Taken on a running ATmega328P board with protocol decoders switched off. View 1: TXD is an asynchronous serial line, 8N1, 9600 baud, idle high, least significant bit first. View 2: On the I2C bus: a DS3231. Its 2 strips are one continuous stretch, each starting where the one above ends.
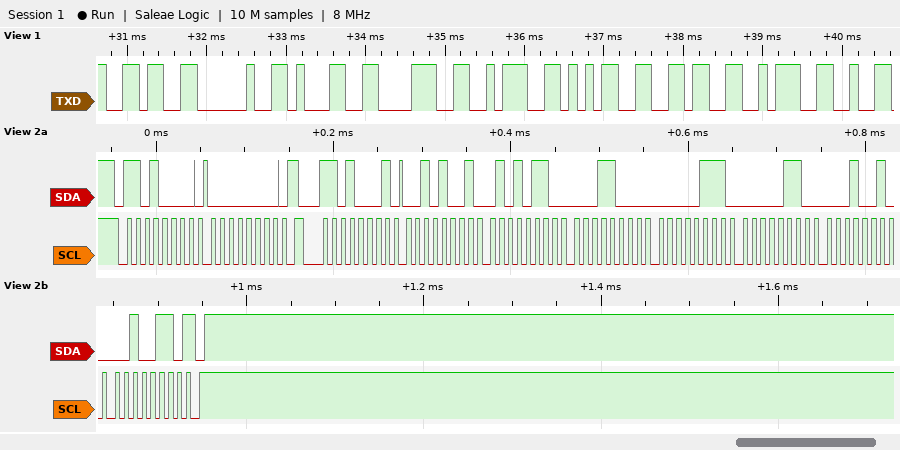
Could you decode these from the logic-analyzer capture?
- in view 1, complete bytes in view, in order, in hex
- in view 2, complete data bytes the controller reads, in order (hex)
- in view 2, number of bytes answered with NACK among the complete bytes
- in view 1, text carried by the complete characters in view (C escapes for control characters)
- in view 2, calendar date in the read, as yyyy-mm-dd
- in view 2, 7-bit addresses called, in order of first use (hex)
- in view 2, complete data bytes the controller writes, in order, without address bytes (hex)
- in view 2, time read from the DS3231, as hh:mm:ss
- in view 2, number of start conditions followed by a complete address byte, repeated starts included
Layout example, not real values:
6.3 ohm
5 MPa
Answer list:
36 20 31 38 3A 35 36 3A
29 56 18 07 06 12 26
1
"6 18:56:"
2026-12-06
0x68
00
18:56:29
2
